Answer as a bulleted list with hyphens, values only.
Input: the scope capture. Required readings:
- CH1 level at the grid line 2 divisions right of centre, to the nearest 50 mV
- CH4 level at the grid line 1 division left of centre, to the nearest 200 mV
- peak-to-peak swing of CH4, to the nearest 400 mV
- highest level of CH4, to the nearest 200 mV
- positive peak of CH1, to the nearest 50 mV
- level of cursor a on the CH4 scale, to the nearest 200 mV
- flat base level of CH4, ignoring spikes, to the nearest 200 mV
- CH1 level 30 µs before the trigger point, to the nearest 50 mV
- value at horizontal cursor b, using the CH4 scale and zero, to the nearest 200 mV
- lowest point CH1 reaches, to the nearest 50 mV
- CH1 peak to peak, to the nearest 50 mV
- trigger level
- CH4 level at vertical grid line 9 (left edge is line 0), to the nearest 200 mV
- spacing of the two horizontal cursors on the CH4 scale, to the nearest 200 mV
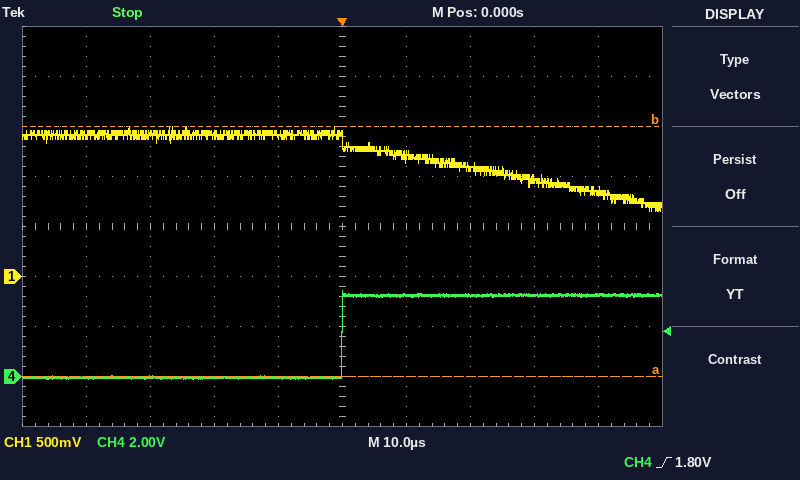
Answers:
- 1.10 V
- 0.0 V
- 3.6 V
- 3.4 V
- 1.50 V
- 0.0 V
- 0.0 V
- 1.40 V
- 10.0 V
- 650 mV
- 850 mV
- 1.80 V
- 3.2 V
- 10.0 V
